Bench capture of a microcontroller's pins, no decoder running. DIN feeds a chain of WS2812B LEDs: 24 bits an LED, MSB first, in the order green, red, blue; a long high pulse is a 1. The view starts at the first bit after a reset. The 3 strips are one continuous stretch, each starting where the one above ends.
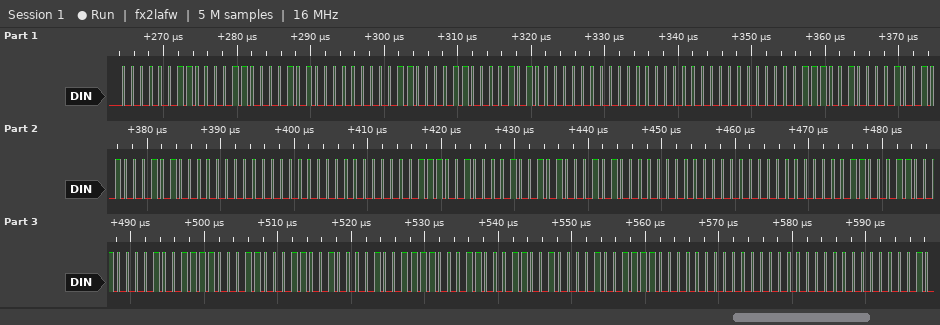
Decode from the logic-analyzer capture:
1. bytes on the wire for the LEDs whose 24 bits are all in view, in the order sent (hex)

03 0C 28 03 0C 28 00 00 00 39 09 45 00 00 00 39 09 45 00 00 00 63 21 3C 63 21 3C 63 21 3C 00 00 00
